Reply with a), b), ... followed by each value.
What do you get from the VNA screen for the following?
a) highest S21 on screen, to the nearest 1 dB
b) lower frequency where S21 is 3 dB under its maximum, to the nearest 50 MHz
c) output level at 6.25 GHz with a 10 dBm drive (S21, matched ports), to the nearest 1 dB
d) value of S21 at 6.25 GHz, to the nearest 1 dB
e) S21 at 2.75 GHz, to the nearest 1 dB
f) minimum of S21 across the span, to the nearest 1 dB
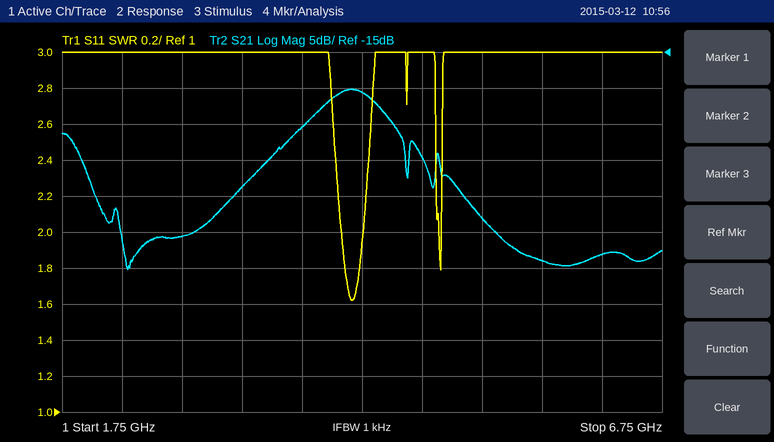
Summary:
a) -20 dB
b) 3.90 GHz
c) -33 dBm
d) -43 dB
e) -41 dB
f) -45 dB
